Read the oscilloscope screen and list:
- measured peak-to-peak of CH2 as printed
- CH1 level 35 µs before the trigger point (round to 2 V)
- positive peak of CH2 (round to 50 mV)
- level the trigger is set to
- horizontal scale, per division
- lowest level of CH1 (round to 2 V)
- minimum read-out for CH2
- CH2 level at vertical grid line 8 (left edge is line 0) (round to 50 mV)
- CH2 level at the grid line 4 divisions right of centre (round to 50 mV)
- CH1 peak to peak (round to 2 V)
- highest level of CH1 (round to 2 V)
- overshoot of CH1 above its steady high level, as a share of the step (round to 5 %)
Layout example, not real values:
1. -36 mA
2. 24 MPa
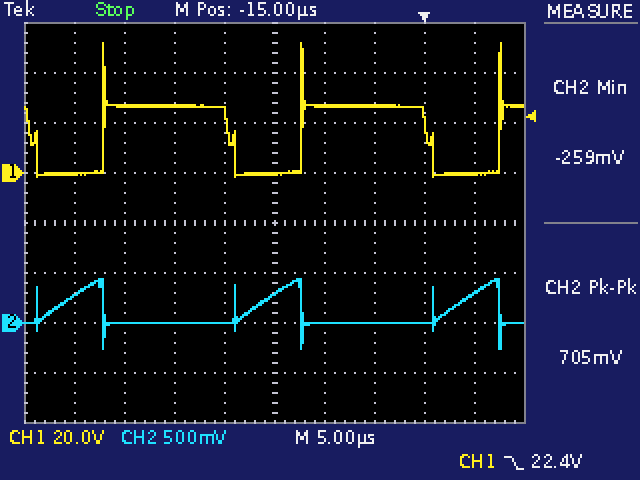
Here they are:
1. 705 mV
2. 0 V
3. 450 mV
4. 22.4 V
5. 5 µs
6. -2 V
7. -259 mV
8. 0 mV
9. 300 mV
10. 54 V
11. 52 V
12. 95 %
